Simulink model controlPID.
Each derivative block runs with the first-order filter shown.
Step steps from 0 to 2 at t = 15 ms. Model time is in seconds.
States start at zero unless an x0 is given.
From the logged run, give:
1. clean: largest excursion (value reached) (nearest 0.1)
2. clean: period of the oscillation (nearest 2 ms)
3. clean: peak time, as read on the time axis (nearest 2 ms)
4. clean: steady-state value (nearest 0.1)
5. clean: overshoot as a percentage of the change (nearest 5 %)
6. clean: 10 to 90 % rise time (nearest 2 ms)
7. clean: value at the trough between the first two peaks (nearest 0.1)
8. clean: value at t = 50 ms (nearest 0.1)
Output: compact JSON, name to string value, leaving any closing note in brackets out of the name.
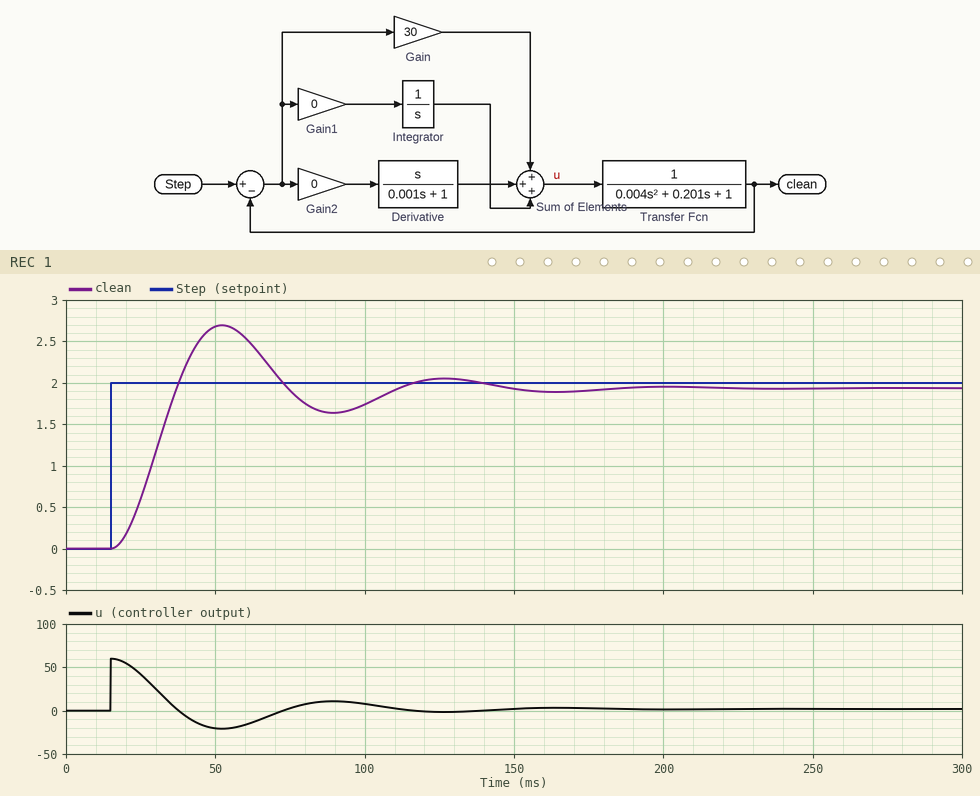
{"clean: largest excursion (value reached)": "2.7", "clean: period of the oscillation": "74 ms", "clean: peak time, as read on the time axis": "52 ms", "clean: steady-state value": "1.9", "clean: overshoot as a percentage of the change": "40 %", "clean: 10 to 90 % rise time": "14 ms", "clean: value at the trough between the first two peaks": "1.6", "clean: value at t = 50 ms": "2.7"}
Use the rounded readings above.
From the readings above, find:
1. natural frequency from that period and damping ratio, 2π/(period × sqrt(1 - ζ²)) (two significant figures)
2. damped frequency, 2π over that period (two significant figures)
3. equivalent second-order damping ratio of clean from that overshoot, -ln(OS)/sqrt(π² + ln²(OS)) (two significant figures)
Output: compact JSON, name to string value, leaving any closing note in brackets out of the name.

{"natural frequency from that period and damping ratio, 2π/(period × sqrt(1 - ζ²))": "0.088 rad/ms", "damped frequency, 2π over that period": "0.085 rad/ms", "equivalent second-order damping ratio of clean from that overshoot, -ln(OS)/sqrt(π² + ln²(OS))": "0.28"}
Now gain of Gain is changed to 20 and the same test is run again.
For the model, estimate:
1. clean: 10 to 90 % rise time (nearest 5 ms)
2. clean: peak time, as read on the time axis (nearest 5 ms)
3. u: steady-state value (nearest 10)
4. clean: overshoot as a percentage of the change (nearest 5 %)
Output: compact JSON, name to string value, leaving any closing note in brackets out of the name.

{"clean: 10 to 90 % rise time": "20 ms", "clean: peak time, as read on the time axis": "60 ms", "u: steady-state value": "0", "clean: overshoot as a percentage of the change": "30 %"}
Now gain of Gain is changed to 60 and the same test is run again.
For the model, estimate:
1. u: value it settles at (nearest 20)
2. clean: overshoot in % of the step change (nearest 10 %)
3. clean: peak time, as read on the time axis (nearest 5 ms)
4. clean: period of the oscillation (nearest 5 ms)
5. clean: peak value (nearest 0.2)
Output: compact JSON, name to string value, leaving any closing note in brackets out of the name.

{"u: value it settles at": "0", "clean: overshoot in % of the step change": "50 %", "clean: peak time, as read on the time axis": "40 ms", "clean: period of the oscillation": "50 ms", "clean: peak value": "3.0"}
